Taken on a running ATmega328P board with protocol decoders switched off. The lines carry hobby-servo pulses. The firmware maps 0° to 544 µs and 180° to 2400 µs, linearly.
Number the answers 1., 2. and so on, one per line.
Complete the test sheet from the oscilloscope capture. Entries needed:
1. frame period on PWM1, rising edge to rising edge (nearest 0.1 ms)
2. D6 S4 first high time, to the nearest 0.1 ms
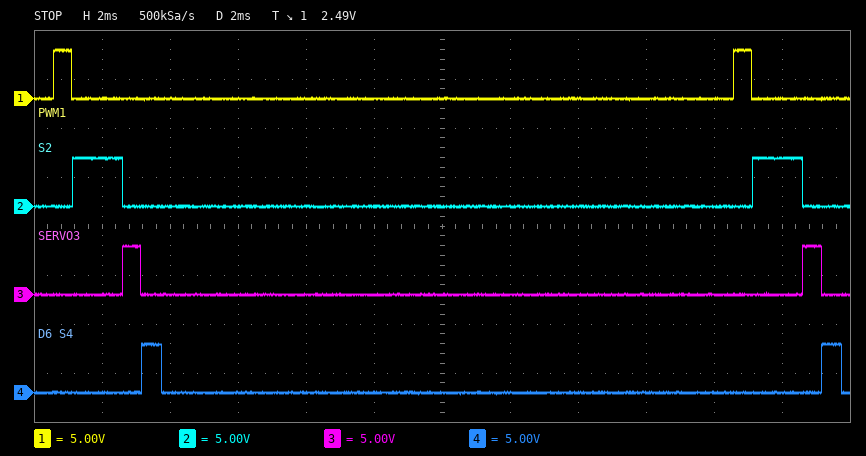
1. 20.0 ms
2. 0.6 ms
